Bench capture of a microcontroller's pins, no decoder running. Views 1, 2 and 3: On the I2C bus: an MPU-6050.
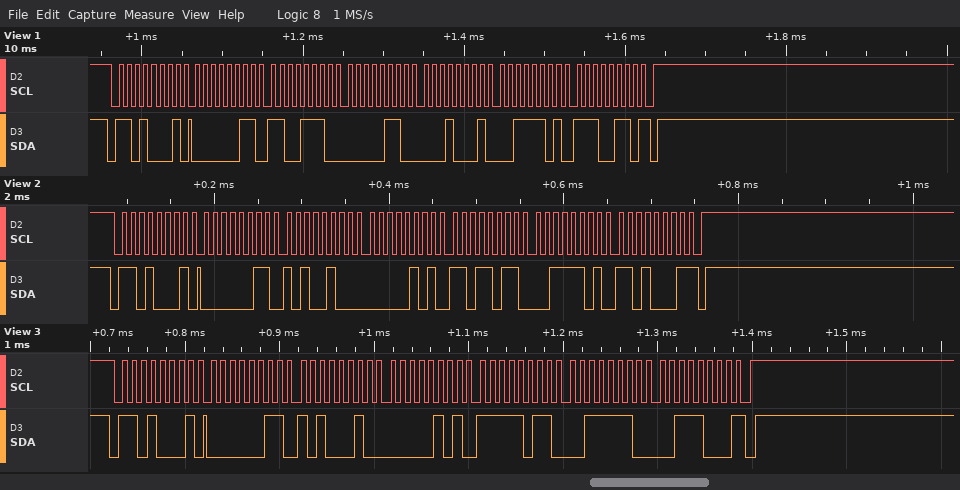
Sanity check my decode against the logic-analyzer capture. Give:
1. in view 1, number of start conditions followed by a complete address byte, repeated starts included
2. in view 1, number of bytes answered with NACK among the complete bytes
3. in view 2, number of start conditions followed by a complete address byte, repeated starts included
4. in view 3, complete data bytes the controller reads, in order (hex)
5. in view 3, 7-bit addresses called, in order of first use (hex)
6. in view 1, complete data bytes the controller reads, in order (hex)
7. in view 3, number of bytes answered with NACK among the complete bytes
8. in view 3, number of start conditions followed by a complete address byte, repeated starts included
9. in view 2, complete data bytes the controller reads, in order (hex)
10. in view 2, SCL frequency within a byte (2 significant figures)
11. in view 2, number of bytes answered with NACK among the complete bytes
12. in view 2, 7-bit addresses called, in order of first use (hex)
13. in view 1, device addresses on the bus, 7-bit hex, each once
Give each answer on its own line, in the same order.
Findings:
1
1
1
03 A2 05 FB 3E 38
0x68
03 CE 06 11 3D E6
1
1
03 A4 05 DB 3D D1
100 kHz
1
0x68
0x68
